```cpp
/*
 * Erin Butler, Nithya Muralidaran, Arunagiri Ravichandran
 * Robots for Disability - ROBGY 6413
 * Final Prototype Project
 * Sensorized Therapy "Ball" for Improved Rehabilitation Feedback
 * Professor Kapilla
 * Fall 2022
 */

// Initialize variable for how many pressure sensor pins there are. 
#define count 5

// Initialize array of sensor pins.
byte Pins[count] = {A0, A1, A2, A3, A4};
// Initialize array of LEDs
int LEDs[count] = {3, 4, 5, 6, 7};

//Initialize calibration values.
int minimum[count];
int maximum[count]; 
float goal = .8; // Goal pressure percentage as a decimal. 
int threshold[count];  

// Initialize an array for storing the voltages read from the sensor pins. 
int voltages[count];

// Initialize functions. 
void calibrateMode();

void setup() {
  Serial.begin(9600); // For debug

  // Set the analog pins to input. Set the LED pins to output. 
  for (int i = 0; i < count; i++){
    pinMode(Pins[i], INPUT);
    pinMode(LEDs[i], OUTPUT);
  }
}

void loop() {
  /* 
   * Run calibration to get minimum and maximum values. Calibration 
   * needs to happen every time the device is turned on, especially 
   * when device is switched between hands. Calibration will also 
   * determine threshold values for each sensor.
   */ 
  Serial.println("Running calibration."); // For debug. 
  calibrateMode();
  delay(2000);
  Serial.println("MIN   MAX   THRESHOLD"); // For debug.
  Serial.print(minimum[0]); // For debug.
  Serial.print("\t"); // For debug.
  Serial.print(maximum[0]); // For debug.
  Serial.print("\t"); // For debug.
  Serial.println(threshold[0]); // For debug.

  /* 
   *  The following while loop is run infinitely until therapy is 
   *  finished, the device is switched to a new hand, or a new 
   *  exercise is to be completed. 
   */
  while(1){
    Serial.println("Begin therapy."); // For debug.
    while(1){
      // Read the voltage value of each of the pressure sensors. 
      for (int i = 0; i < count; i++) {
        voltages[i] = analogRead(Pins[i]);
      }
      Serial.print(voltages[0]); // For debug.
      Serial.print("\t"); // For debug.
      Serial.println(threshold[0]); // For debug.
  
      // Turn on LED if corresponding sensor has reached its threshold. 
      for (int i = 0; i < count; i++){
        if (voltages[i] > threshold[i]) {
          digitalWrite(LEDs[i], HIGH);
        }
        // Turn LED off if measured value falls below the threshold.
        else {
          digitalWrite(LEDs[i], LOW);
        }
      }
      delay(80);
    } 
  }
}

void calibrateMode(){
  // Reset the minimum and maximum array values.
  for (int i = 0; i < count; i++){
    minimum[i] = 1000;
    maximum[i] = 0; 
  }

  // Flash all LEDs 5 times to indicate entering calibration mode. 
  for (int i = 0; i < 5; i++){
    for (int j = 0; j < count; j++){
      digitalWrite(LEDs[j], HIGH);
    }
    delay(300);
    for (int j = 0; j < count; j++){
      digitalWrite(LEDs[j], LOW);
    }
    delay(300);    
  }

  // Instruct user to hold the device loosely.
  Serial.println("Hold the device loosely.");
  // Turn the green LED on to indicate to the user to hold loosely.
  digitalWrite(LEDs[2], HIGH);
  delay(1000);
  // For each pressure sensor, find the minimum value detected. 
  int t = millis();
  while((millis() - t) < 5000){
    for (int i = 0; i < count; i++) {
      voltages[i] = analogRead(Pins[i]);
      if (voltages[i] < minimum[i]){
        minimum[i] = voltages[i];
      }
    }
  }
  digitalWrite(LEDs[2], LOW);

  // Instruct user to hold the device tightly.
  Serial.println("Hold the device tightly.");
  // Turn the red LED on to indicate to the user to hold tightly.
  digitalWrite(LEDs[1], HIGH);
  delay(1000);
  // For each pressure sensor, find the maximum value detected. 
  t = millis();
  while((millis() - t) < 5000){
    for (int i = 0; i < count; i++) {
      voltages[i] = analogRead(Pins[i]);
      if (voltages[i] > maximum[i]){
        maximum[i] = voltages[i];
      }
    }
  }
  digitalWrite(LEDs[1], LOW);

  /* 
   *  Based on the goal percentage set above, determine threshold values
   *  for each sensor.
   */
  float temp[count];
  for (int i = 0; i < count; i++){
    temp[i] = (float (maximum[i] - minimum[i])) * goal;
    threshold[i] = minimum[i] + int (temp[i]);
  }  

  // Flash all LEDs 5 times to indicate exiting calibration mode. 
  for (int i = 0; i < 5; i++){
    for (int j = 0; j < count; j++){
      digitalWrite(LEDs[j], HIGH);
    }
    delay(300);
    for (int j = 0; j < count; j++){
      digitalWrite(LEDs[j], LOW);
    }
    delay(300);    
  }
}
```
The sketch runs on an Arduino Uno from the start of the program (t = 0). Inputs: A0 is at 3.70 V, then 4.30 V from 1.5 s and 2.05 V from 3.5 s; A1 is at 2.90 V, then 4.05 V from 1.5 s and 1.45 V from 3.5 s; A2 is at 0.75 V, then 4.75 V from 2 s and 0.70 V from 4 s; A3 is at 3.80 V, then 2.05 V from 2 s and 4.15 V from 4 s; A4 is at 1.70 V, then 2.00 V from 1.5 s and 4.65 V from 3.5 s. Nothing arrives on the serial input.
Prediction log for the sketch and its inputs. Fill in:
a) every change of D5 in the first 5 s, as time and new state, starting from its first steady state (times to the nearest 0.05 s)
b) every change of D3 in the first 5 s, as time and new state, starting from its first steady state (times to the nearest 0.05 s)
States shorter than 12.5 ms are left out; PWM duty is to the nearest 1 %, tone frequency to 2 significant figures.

0 s high; 0.3 s low; 0.6 s high; 0.9 s low; 1.2 s high; 1.5 s low; 1.8 s high; 2.1 s low; 2.4 s high; 2.7 s low; 3 s high
0 s high; 0.3 s low; 0.6 s high; 0.9 s low; 1.2 s high; 1.5 s low; 1.8 s high; 2.1 s low; 2.4 s high; 2.7 s low
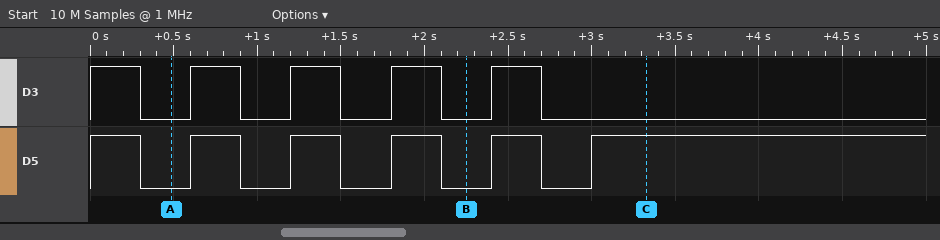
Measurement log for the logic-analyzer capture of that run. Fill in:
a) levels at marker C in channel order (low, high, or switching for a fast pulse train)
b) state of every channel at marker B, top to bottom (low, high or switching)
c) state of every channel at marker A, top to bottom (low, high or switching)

D3 low, D5 high
D3 low, D5 low
D3 low, D5 low
